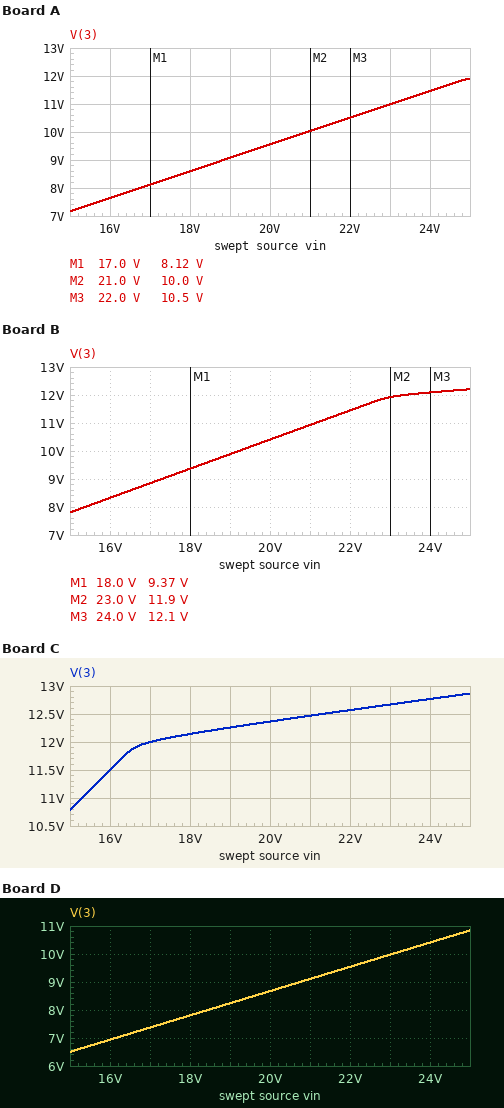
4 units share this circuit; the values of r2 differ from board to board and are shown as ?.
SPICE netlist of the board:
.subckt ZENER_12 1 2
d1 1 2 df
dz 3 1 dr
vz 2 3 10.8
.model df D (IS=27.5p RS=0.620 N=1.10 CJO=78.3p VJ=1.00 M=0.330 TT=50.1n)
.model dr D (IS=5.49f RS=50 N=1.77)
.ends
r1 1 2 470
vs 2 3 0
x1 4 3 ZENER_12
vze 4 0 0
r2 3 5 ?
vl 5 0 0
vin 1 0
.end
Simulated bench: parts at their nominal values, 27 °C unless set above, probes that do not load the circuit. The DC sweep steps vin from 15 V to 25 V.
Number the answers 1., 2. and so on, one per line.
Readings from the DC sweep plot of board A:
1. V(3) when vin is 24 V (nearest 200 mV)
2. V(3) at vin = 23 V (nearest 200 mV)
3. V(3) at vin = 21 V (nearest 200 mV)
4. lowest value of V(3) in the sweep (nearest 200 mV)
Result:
1. 11.4 V
2. 11.0 V
3. 10.0 V
4. 7.2 V
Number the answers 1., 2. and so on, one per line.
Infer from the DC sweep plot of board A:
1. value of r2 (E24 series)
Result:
1. 430 Ω
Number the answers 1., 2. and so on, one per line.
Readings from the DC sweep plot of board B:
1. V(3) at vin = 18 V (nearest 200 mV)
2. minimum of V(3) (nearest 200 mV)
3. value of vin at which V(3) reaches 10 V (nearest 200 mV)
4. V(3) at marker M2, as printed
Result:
1. 9.4 V
2. 7.8 V
3. 19.2 V
4. 11.9 V
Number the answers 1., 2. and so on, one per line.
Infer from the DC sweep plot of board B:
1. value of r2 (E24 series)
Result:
1. 510 Ω
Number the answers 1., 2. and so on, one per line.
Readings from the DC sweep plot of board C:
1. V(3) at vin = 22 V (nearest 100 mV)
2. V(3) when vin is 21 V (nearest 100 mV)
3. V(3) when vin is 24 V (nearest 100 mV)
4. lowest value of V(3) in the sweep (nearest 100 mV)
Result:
1. 12.6 V
2. 12.5 V
3. 12.8 V
4. 10.8 V
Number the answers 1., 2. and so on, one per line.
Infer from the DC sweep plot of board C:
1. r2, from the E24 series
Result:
1. 1.2 kΩ
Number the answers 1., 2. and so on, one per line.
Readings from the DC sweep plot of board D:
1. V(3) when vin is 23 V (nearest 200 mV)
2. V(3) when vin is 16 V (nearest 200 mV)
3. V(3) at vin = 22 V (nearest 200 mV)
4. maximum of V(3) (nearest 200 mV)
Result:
1. 10.0 V
2. 7.0 V
3. 9.6 V
4. 10.8 V
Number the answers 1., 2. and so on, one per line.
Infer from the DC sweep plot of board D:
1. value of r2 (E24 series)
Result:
1. 360 Ω
